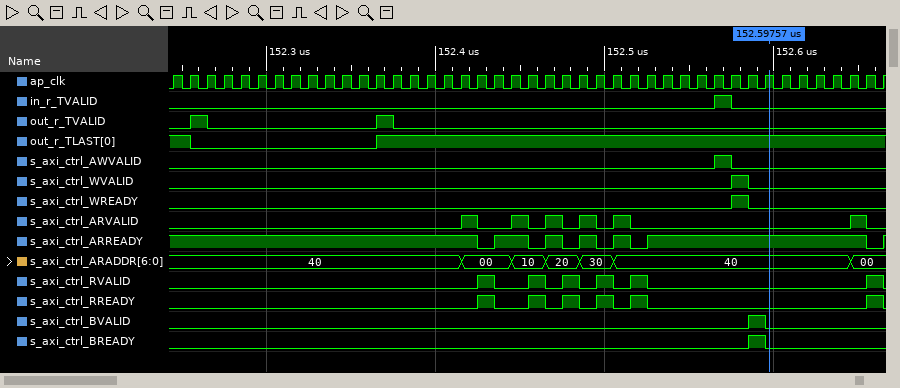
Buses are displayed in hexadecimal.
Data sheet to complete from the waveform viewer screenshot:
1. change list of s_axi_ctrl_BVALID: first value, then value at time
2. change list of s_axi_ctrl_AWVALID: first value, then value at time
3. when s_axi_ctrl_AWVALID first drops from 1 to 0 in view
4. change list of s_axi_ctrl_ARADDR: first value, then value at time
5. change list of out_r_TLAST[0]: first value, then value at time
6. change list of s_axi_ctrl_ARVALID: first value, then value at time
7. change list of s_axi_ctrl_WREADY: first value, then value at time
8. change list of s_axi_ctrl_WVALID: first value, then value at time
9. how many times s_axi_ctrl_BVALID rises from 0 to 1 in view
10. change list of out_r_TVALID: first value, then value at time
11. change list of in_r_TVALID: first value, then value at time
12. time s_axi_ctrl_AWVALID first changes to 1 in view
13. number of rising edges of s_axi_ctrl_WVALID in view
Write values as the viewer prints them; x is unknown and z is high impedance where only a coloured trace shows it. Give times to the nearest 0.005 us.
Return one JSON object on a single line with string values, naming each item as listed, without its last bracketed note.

{"change list of s_axi_ctrl_BVALID: first value, then value at time": "0, 1 at 152.585 us, 0 at 152.595 us", "change list of s_axi_ctrl_AWVALID: first value, then value at time": "0, 1 at 152.565 us, 0 at 152.575 us", "when s_axi_ctrl_AWVALID first drops from 1 to 0 in view": "152.575 us", "change list of s_axi_ctrl_ARADDR: first value, then value at time": "40, 00 at 152.415 us, 10 at 152.445 us, 20 at 152.465 us, 30 at 152.485 us, 40 at 152.505 us, 00 at 152.645 us", "change list of out_r_TLAST[0]: first value, then value at time": "1, 0 at 152.255 us, 1 at 152.365 us", "change list of s_axi_ctrl_ARVALID: first value, then value at time": "0, 1 at 152.415 us, 0 at 152.425 us, 1 at 152.445 us, 0 at 152.455 us, 1 at 152.465 us, 0 at 152.475 us, 1 at 152.485 us, 0 at 152.495 us, 1 at 152.505 us, 0 at 152.515 us, 1 at 152.645 us, 0 at 152.655 us", "change list of s_axi_ctrl_WREADY: first value, then value at time": "0, 1 at 152.575 us, 0 at 152.585 us", "change list of s_axi_ctrl_WVALID: first value, then value at time": "0, 1 at 152.575 us, 0 at 152.585 us", "how many times s_axi_ctrl_BVALID rises from 0 to 1 in view": "1", "change list of out_r_TVALID: first value, then value at time": "0, 1 at 152.255 us, 0 at 152.265 us, 1 at 152.365 us, 0 at 152.375 us", "change list of in_r_TVALID: first value, then value at time": "0, 1 at 152.565 us, 0 at 152.575 us", "time s_axi_ctrl_AWVALID first changes to 1 in view": "152.565 us", "number of rising edges of s_axi_ctrl_WVALID in view": "1"}
